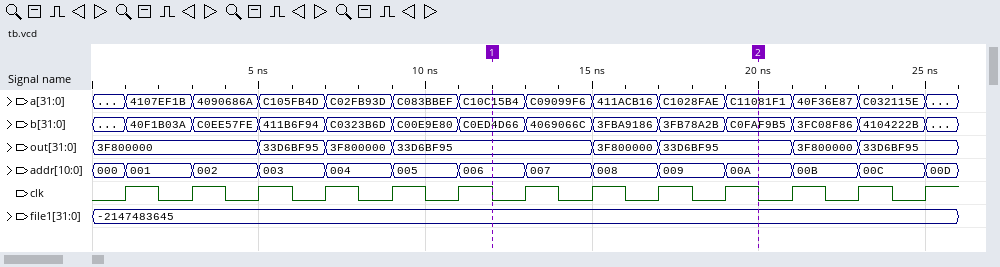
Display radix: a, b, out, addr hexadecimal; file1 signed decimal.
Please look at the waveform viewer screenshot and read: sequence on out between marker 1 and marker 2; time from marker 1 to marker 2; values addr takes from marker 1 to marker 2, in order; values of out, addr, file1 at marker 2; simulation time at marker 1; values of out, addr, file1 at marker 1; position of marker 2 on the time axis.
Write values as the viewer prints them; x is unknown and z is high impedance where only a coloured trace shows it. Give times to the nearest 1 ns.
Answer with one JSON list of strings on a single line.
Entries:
["33D6BF95, 3F800000, 33D6BF95", "8 ns", "006, 007, 008, 009, 00A", "out=33D6BF95, addr=00A, file1=-2147483645", "12 ns", "out=33D6BF95, addr=006, file1=-2147483645", "20 ns"]
